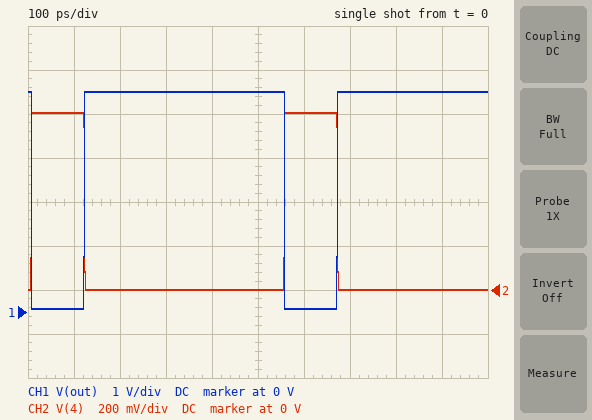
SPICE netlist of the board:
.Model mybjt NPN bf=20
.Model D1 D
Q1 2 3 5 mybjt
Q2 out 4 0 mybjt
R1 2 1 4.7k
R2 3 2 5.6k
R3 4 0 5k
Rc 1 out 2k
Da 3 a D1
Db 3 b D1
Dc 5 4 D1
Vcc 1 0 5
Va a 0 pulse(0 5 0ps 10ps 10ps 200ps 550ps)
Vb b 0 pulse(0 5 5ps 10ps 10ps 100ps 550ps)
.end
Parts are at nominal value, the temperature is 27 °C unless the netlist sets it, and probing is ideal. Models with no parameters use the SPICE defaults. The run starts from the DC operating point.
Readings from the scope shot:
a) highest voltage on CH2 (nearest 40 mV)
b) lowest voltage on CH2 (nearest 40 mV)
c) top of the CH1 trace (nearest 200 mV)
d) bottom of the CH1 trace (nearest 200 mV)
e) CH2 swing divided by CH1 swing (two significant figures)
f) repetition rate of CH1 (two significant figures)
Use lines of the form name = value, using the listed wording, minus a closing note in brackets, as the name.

highest voltage on CH2 = 800 mV
lowest voltage on CH2 = 0 V
top of the CH1 trace = 5.0 V
bottom of the CH1 trace = 0 V
CH2 swing divided by CH1 swing = 0.16
repetition rate of CH1 = 1.8 GHz
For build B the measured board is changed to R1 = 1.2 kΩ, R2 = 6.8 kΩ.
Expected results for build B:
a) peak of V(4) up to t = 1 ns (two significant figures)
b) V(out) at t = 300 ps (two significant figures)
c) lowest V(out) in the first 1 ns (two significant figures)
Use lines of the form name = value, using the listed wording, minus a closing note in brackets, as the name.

peak of V(4) up to t = 1 ns = 820 mV
V(out) at t = 300 ps = 5.0 V
lowest V(out) in the first 1 ns = 35 mV
